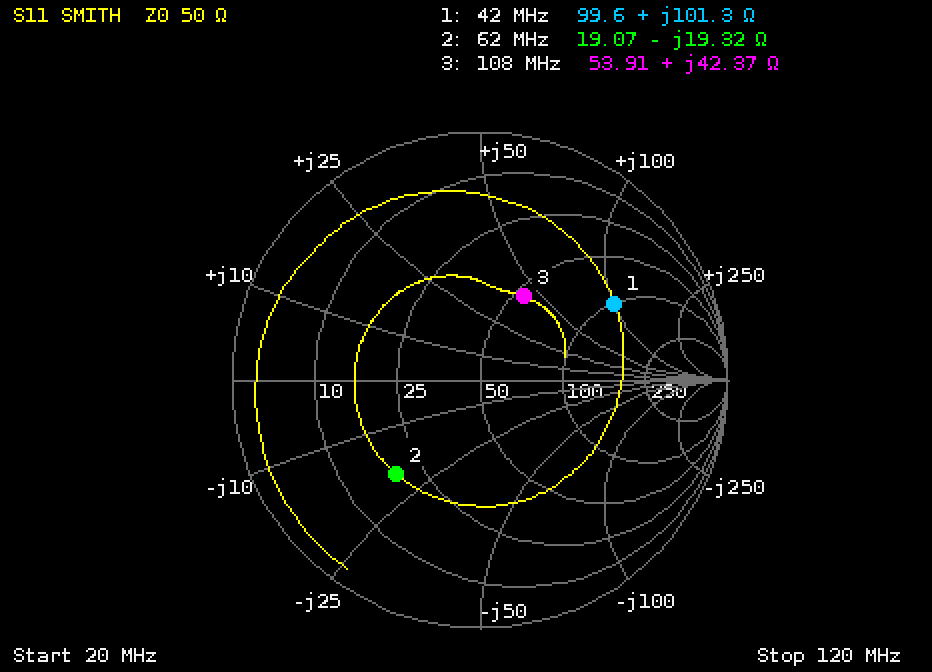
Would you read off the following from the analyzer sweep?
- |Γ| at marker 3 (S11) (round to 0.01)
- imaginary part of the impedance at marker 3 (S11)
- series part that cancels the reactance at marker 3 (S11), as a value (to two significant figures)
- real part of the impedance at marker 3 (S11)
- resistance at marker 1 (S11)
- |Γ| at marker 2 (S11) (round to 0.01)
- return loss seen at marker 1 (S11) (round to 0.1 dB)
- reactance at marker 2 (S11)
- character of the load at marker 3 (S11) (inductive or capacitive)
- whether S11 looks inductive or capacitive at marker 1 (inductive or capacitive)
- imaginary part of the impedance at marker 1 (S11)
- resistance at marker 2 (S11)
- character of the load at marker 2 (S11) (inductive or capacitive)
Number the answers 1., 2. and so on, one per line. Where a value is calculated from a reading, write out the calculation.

1. 0.38
2. +42.37 Ω
3. C = 1/(2π × 108 MHz × 42.37 Ω) ≈ 35 pF
4. 53.91 Ω
5. 99.6 Ω
6. 0.51
7. 4.1 dB
8. -19.32 Ω
9. inductive
10. inductive
11. +101.3 Ω
12. 19.07 Ω
13. capacitive
